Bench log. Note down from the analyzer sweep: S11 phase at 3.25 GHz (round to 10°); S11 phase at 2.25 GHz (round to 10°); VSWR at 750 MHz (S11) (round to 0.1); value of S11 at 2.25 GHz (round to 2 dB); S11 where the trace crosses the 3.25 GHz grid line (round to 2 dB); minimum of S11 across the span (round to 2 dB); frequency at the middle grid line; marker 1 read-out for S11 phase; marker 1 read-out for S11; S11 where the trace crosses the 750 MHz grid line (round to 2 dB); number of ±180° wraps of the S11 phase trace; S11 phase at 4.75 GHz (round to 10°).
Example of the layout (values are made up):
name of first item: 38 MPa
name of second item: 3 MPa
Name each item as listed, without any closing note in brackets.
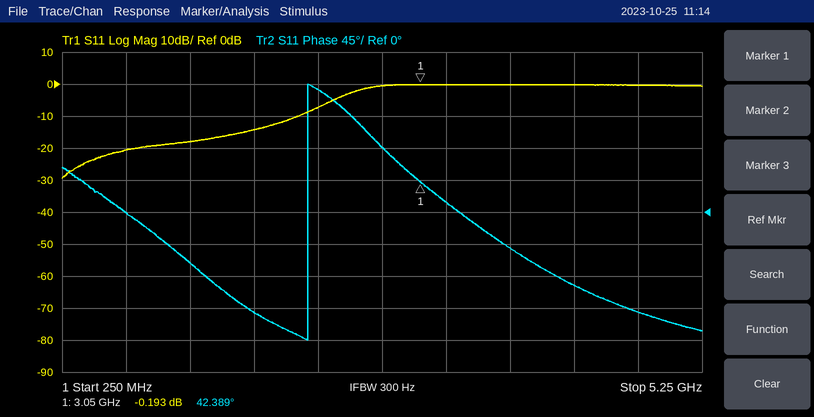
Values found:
S11 phase at 3.25 GHz: 10°
S11 phase at 2.25 GHz: 170°
VSWR at 750 MHz (S11): 1.2
value of S11 at 2.25 GHz: -8 dB
S11 where the trace crosses the 3.25 GHz grid line: 0 dB
minimum of S11 across the span: -30 dB
frequency at the middle grid line: 2.75 GHz
marker 1 read-out for S11 phase: 42.389°
marker 1 read-out for S11: -0.193 dB
S11 where the trace crosses the 750 MHz grid line: -20 dB
number of ±180° wraps of the S11 phase trace: 1
S11 phase at 4.75 GHz: -140°
